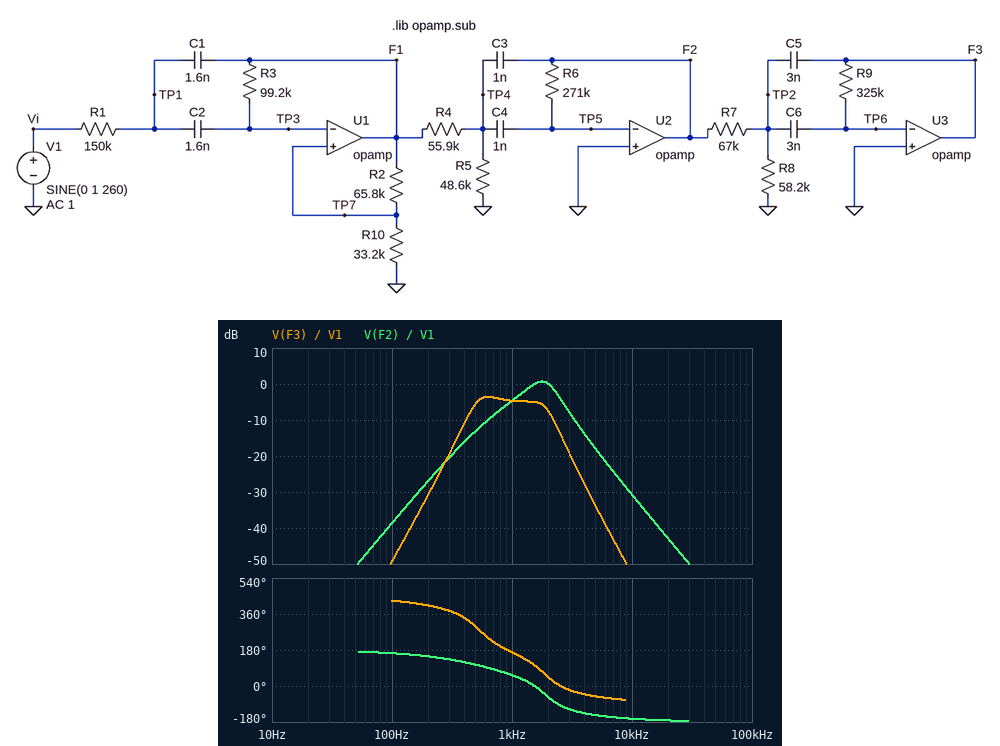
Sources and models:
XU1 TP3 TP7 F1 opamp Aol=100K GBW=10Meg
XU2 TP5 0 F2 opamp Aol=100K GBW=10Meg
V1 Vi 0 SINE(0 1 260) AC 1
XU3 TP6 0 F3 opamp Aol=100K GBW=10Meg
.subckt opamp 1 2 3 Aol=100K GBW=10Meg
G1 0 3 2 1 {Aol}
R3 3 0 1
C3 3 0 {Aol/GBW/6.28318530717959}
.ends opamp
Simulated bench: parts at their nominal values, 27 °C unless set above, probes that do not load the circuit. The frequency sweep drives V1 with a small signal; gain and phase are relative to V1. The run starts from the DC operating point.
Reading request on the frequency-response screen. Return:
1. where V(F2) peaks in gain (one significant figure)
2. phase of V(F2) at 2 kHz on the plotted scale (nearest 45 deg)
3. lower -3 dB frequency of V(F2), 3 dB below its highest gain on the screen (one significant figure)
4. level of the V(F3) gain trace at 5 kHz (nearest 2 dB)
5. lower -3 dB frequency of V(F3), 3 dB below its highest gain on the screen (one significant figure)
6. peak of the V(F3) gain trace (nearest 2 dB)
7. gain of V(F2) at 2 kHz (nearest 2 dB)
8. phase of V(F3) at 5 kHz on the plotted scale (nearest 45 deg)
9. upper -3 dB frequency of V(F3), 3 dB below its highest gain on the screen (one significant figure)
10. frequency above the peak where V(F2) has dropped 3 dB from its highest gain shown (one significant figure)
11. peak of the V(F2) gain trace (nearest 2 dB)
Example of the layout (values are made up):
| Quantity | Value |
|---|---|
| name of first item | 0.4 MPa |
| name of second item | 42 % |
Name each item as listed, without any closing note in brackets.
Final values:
| Quantity | Value |
|---|---|
| where V(F2) peaks in gain | 2 kHz |
| phase of V(F2) at 2 kHz on the plotted scale | -45 deg |
| lower -3 dB frequency of V(F2), 3 dB below its highest gain on the screen | 1 kHz |
| level of the V(F3) gain trace at 5 kHz | -34 dB |
| lower -3 dB frequency of V(F3), 3 dB below its highest gain on the screen | 500 Hz |
| peak of the V(F3) gain trace | -4 dB |
| gain of V(F2) at 2 kHz | 0 dB |
| phase of V(F3) at 5 kHz on the plotted scale | -45 deg |
| upper -3 dB frequency of V(F3), 3 dB below its highest gain on the screen | 2 kHz |
| frequency above the peak where V(F2) has dropped 3 dB from its highest gain shown | 2 kHz |
| peak of the V(F2) gain trace | 0 dB |
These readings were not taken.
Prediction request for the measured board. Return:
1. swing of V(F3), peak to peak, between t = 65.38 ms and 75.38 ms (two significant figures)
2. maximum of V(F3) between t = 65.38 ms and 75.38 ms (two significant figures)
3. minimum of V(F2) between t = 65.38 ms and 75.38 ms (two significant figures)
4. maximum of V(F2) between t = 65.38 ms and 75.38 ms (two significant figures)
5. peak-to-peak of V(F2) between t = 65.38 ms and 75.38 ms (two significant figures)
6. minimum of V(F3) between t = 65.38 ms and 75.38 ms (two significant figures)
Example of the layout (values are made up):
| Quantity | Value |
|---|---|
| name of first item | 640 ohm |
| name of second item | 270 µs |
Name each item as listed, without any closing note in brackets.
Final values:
| Quantity | Value |
|---|---|
| swing of V(F3), peak to peak, between t = 65.38 ms and 75.38 ms | 130 mV |
| maximum of V(F3) between t = 65.38 ms and 75.38 ms | 67 mV |
| minimum of V(F2) between t = 65.38 ms and 75.38 ms | -73 mV |
| maximum of V(F2) between t = 65.38 ms and 75.38 ms | 73 mV |
| peak-to-peak of V(F2) between t = 65.38 ms and 75.38 ms | 150 mV |
| minimum of V(F3) between t = 65.38 ms and 75.38 ms | -67 mV |
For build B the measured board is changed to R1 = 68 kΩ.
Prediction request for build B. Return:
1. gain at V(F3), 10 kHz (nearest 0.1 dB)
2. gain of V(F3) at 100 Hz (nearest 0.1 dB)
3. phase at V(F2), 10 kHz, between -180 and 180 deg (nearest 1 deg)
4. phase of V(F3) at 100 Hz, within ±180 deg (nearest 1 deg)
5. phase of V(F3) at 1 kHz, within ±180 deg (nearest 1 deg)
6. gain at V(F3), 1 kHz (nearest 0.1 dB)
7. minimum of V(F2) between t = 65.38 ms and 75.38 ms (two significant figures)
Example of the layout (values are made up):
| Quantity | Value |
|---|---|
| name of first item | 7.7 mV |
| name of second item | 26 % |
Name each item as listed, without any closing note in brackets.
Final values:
| Quantity | Value |
|---|---|
| gain at V(F3), 10 kHz | -45.8 dB |
| gain of V(F3) at 100 Hz | -49.1 dB |
| phase at V(F2), 10 kHz, between -180 and 180 deg | -166 deg |
| phase of V(F3) at 100 Hz, within ±180 deg | 76 deg |
| phase of V(F3) at 1 kHz, within ±180 deg | -160 deg |
| gain at V(F3), 1 kHz | 4.2 dB |
| minimum of V(F2) between t = 65.38 ms and 75.38 ms | -83 mV |
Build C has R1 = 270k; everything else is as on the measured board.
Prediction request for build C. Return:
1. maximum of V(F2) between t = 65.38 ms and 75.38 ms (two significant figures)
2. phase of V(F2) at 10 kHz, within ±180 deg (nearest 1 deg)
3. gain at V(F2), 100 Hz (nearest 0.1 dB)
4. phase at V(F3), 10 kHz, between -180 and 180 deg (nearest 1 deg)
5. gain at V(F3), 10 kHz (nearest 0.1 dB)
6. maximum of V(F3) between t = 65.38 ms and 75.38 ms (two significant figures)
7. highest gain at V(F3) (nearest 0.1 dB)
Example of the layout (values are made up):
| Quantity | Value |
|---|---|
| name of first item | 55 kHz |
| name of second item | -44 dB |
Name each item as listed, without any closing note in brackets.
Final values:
| Quantity | Value |
|---|---|
| maximum of V(F2) between t = 65.38 ms and 75.38 ms | 54 mV |
| phase of V(F2) at 10 kHz, within ±180 deg | -163 deg |
| gain at V(F2), 100 Hz | -39.2 dB |
| phase at V(F3), 10 kHz, between -180 and 180 deg | -71 deg |
| gain at V(F3), 10 kHz | -57.9 dB |
| maximum of V(F3) between t = 65.38 ms and 75.38 ms | 49 mV |
| highest gain at V(F3) | -9.1 dB |
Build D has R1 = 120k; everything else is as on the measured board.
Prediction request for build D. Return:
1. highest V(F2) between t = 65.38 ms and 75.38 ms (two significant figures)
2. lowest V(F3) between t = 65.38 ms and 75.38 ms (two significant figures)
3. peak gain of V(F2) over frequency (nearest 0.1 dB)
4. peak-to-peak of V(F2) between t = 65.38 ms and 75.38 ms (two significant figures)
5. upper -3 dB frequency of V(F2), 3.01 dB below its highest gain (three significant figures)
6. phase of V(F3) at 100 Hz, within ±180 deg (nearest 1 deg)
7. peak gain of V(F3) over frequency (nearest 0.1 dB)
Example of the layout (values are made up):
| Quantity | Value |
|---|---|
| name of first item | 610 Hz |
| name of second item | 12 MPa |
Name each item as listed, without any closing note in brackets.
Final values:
| Quantity | Value |
|---|---|
| highest V(F2) between t = 65.38 ms and 75.38 ms | 78 mV |
| lowest V(F3) between t = 65.38 ms and 75.38 ms | -71 mV |
| peak gain of V(F2) over frequency | 3.2 dB |
| peak-to-peak of V(F2) between t = 65.38 ms and 75.38 ms | 160 mV |
| upper -3 dB frequency of V(F2), 3.01 dB below its highest gain | 2.30 kHz |
| phase of V(F3) at 100 Hz, within ±180 deg | 70 deg |
| peak gain of V(F3) over frequency | -1.6 dB |
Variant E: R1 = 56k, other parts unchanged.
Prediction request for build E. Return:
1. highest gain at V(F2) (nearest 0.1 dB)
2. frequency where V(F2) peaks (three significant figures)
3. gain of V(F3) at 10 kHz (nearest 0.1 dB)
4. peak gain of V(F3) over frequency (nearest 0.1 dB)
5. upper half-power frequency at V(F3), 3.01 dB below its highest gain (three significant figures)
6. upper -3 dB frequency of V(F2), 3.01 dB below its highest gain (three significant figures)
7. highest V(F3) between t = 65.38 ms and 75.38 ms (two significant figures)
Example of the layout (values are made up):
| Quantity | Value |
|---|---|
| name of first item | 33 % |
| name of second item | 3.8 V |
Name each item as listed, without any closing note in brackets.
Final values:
| Quantity | Value |
|---|---|
| highest gain at V(F2) | 13.5 dB |
| frequency where V(F2) peaks | 1.69 kHz |
| gain of V(F3) at 10 kHz | -44.0 dB |
| peak gain of V(F3) over frequency | 8.4 dB |
| upper half-power frequency at V(F3), 3.01 dB below its highest gain | 1.94 kHz |
| upper -3 dB frequency of V(F2), 3.01 dB below its highest gain | 2.18 kHz |
| highest V(F3) between t = 65.38 ms and 75.38 ms | 76 mV |
